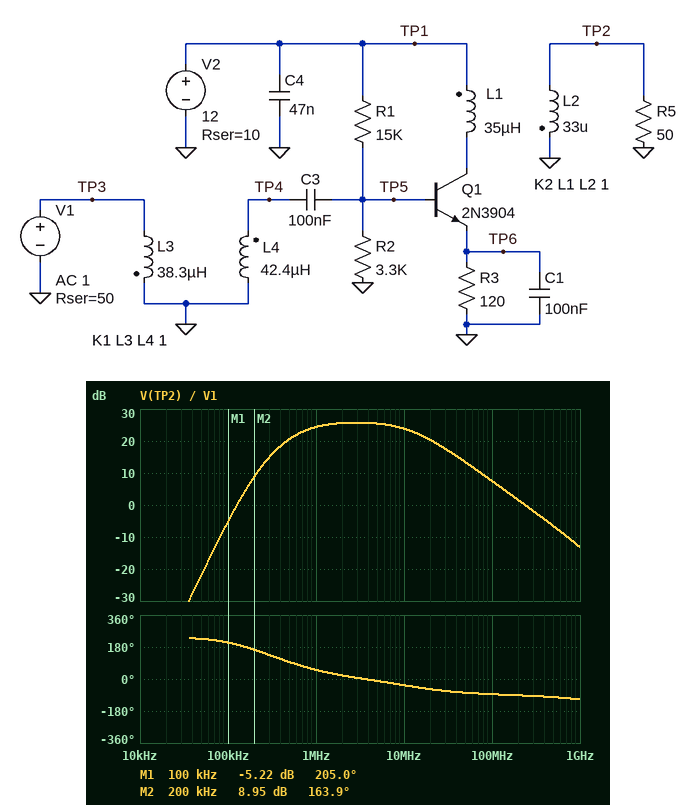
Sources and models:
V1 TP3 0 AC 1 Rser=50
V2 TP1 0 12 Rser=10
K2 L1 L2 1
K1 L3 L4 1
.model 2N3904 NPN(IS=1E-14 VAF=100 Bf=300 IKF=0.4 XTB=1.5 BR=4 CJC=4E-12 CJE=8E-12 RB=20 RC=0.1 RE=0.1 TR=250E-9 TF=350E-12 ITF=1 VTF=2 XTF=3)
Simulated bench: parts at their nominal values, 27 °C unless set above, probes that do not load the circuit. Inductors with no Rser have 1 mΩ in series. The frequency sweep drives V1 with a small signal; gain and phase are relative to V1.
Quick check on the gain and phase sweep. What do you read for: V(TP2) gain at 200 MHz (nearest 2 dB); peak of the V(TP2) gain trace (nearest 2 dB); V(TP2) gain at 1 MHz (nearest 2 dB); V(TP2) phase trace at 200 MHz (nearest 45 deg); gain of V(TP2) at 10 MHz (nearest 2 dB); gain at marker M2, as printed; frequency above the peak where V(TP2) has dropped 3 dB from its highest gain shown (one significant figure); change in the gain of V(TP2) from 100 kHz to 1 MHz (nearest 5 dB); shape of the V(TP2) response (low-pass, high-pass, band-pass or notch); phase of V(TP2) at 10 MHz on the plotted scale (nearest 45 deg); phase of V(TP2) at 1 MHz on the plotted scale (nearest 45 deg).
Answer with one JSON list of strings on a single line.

["2 dB", "26 dB", "24 dB", "-90 deg", "24 dB", "8.95 dB", "10 MHz", "30 dB", "band-pass", "-45 deg", "45 deg"]
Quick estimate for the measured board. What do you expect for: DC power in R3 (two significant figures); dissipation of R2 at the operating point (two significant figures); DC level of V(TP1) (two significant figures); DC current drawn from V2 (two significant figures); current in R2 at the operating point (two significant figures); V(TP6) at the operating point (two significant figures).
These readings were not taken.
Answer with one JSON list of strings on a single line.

["15 mW", "1.3 mW", "12 V", "12 mA", "620 µA", "1.3 V"]
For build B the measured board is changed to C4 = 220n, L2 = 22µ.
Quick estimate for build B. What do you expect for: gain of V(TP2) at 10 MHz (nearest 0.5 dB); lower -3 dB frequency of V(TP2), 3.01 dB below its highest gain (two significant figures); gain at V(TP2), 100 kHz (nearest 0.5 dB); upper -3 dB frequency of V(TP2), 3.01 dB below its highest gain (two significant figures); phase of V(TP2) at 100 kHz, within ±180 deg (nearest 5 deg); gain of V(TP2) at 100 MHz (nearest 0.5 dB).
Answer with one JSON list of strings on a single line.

["25.5 dB", "740 kHz", "-6.5 dB", "12 MHz", "-150 deg", "8.5 dB"]
